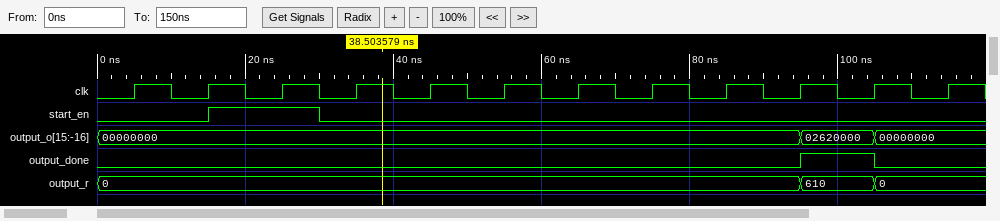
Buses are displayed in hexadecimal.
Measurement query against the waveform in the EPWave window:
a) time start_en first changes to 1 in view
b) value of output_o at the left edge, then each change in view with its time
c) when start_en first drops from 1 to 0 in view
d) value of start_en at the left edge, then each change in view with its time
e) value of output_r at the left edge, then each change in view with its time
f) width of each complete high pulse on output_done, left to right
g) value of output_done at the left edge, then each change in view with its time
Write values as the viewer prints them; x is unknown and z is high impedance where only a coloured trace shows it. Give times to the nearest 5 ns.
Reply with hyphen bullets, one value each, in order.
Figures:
- 15 ns
- 00000000, 02620000 at 95 ns, 00000000 at 105 ns
- 30 ns
- 0, 1 at 15 ns, 0 at 30 ns
- 0, 610 at 95 ns, 0 at 105 ns
- 10 ns
- 0, 1 at 95 ns, 0 at 105 ns
